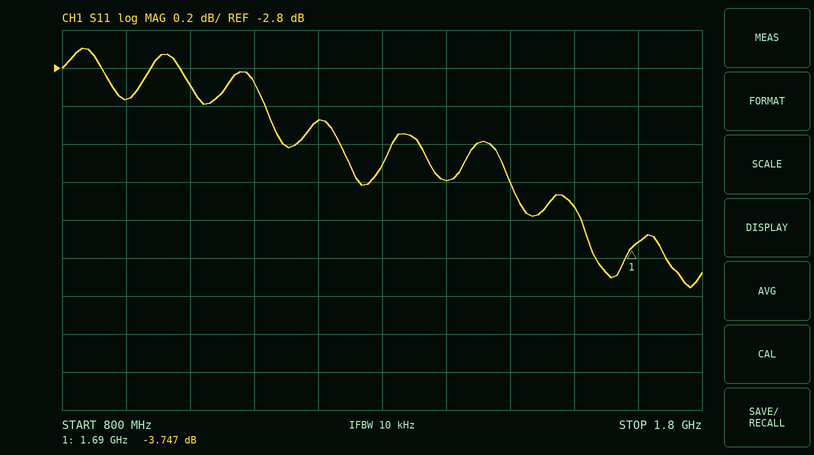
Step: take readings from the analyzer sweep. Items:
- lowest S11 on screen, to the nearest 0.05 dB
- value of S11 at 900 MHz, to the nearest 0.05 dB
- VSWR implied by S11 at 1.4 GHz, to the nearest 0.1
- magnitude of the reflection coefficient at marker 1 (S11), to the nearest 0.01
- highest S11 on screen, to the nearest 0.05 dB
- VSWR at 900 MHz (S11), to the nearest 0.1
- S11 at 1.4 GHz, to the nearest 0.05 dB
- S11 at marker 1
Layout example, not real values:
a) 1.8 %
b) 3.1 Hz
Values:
a) -3.95 dB
b) -2.95 dB
c) 5.2
d) 0.65
e) -2.70 dB
f) 5.9
g) -3.40 dB
h) -3.747 dB
